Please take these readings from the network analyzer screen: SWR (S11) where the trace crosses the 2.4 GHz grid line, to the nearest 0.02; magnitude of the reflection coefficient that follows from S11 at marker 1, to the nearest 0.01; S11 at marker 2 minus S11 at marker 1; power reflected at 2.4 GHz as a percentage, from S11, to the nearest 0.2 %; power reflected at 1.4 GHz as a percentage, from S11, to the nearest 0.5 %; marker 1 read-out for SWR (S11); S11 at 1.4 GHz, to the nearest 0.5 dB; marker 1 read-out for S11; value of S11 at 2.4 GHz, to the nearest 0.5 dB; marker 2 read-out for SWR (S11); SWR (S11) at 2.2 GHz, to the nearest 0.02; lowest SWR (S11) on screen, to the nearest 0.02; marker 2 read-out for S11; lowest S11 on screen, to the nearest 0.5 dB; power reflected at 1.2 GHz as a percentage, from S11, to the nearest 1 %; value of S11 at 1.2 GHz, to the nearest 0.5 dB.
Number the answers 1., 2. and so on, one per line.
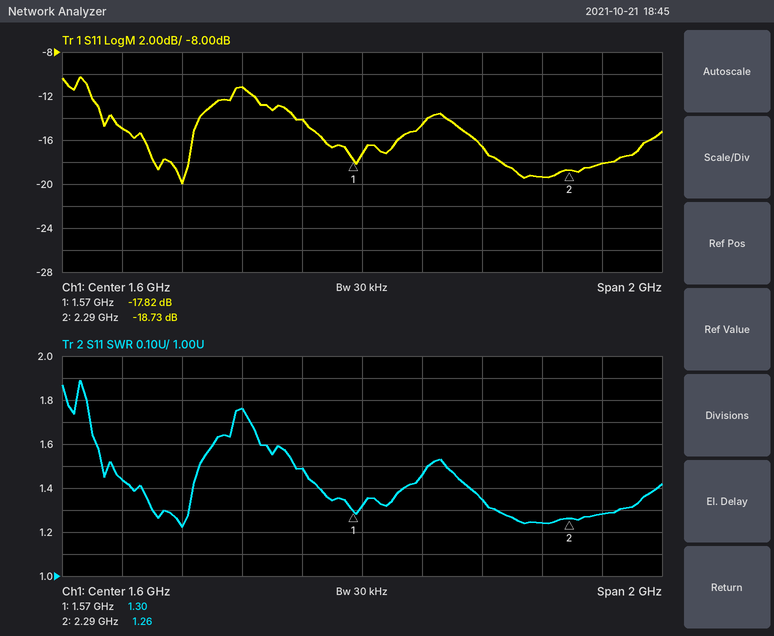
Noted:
1. 1.28
2. 0.13
3. -0.91 dB
4. 1.6 %
5. 4.0 %
6. 1.30
7. -14.0 dB
8. -17.82 dB
9. -18.0 dB
10. 1.26
11. 1.24
12. 1.22
13. -18.73 dB
14. -20.0 dB
15. 8 %
16. -11.0 dB
